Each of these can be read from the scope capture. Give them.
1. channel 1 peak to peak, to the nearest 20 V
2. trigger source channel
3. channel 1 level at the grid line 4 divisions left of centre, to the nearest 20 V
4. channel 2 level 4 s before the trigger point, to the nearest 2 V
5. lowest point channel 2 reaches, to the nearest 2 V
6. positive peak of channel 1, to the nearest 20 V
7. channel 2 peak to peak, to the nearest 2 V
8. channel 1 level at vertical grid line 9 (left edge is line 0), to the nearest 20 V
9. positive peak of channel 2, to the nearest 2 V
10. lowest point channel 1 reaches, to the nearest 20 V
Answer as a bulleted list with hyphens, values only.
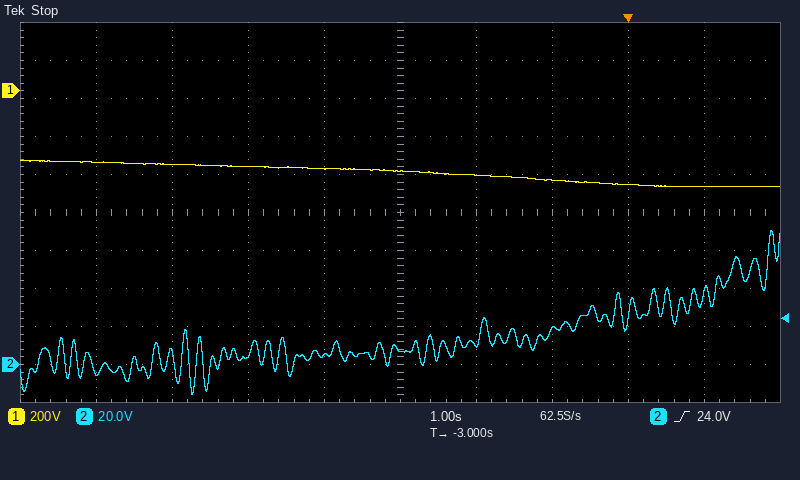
- 140 V
- channel 2
- -380 V
- 4 V
- -16 V
- -360 V
- 86 V
- -500 V
- 70 V
- -500 V
